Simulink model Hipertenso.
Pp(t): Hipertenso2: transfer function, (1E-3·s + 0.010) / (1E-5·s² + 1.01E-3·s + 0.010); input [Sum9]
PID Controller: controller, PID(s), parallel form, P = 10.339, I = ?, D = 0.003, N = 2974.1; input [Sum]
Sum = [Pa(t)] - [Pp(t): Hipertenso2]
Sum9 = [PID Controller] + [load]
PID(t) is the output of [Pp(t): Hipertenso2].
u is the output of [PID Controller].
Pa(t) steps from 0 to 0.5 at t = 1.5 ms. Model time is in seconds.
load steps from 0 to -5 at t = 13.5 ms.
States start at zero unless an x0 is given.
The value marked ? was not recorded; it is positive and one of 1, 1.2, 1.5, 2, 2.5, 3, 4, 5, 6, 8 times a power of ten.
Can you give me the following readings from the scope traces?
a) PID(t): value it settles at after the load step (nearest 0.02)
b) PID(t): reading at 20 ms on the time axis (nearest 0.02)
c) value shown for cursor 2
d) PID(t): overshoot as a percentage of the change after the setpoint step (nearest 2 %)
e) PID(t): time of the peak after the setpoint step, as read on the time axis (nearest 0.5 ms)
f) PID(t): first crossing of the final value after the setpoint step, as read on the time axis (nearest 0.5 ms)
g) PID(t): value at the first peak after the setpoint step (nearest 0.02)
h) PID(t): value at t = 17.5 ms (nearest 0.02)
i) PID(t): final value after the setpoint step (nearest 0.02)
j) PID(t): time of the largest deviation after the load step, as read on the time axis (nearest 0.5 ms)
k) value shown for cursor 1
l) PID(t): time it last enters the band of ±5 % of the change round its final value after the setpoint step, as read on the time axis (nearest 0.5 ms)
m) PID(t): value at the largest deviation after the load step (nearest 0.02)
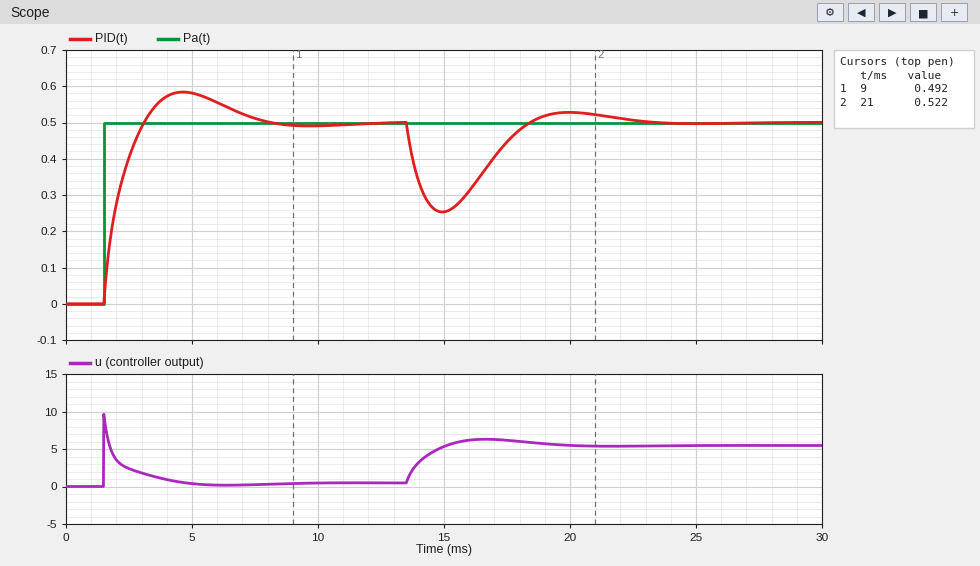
0.50
0.52
0.522
16 %
4.5 ms
3.0 ms
0.58
0.44
0.50
15.0 ms
0.492
7.0 ms
0.26
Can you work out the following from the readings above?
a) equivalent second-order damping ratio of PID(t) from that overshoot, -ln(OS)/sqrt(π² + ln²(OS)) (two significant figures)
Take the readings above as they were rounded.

0.50
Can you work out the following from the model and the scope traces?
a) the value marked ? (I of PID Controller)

8000
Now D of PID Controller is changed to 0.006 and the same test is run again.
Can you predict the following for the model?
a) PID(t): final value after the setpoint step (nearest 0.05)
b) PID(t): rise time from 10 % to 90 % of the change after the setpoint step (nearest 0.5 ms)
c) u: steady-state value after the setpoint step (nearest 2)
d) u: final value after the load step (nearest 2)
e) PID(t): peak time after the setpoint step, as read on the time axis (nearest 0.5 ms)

0.50
1.5 ms
0
6
5.0 ms
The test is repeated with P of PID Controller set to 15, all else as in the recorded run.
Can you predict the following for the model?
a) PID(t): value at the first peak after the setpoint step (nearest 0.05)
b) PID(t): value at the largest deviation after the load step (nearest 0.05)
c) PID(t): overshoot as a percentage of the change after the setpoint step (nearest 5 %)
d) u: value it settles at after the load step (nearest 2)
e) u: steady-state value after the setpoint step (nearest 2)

0.55
0.30
10 %
6
0
